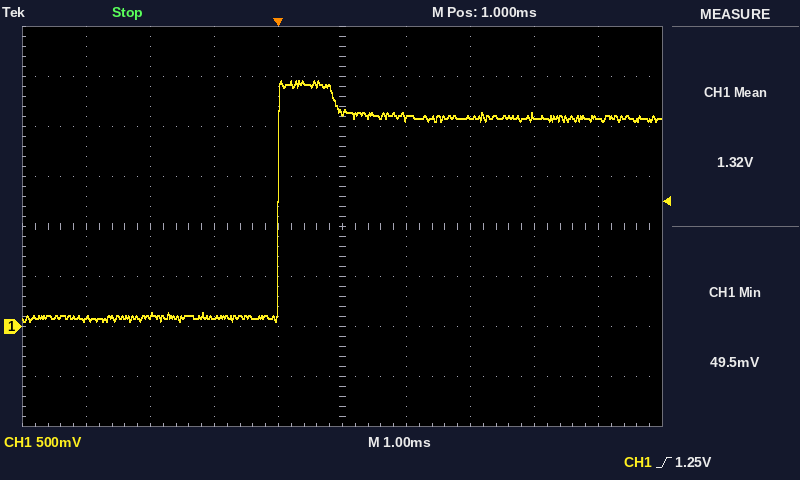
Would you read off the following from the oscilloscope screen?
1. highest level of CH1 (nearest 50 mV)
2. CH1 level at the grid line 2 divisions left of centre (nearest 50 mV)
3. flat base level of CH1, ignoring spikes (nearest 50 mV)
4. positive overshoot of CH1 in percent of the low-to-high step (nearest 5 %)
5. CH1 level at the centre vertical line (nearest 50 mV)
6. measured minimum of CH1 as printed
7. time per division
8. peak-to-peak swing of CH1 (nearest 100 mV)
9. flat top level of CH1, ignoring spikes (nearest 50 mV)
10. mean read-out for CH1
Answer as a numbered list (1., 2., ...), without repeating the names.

1. 2.45 V
2. 100 mV
3. 100 mV
4. 20 %
5. 2.15 V
6. 49.5 mV
7. 1 ms
8. 2.40 V
9. 2.10 V
10. 1.32 V
